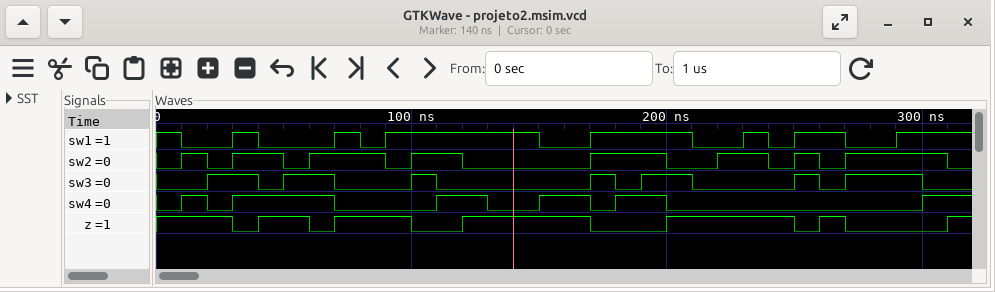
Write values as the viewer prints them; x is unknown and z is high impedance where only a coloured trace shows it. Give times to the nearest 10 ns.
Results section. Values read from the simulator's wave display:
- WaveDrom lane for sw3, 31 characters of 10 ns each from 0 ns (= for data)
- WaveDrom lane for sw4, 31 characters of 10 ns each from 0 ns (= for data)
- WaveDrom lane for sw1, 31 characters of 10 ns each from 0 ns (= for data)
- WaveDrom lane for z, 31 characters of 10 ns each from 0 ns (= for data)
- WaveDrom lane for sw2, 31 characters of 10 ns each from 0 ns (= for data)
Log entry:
{name: 'sw3', wave: '0.1.01.0..10.....101.0...101..0'}
{name: 'sw4', wave: '0101...0...1.0.1.01.0.........1'}
{name: 'sw1', wave: '10.10..101.....0.1...0.101.0.1.'}
{name: 'z', wave: '1..01.01..0.1....0..1....010...'}
{name: 'sw2', wave: '0101.01..01.0....1..0.1.0101...'}
